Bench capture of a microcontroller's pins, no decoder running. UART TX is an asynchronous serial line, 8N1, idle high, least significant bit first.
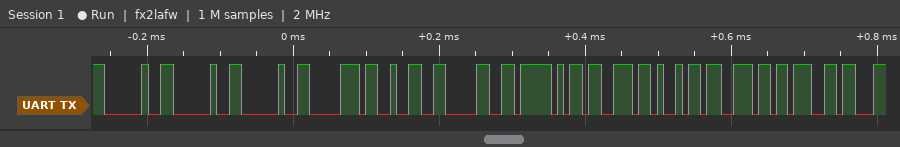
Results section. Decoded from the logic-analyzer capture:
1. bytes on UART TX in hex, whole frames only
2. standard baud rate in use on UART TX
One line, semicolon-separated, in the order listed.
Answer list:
0x20 0x20 0x20 0x70 0x32 0x30 0x5F 0x73 0x69 0x6E 0x67; 115200 baud
